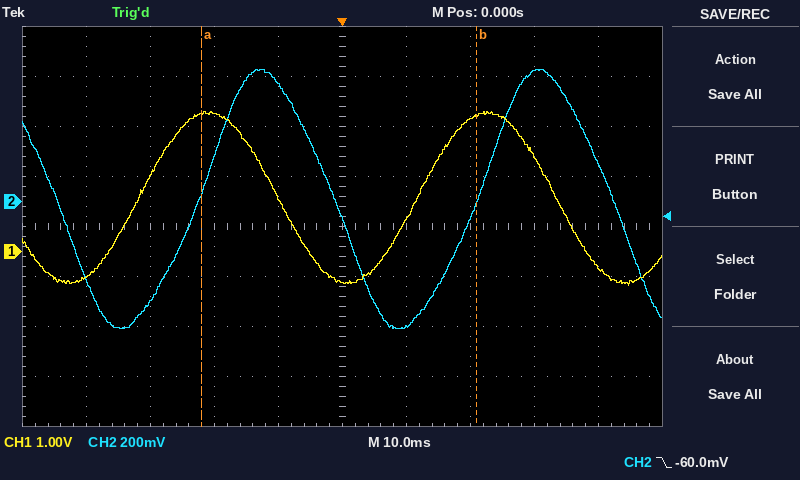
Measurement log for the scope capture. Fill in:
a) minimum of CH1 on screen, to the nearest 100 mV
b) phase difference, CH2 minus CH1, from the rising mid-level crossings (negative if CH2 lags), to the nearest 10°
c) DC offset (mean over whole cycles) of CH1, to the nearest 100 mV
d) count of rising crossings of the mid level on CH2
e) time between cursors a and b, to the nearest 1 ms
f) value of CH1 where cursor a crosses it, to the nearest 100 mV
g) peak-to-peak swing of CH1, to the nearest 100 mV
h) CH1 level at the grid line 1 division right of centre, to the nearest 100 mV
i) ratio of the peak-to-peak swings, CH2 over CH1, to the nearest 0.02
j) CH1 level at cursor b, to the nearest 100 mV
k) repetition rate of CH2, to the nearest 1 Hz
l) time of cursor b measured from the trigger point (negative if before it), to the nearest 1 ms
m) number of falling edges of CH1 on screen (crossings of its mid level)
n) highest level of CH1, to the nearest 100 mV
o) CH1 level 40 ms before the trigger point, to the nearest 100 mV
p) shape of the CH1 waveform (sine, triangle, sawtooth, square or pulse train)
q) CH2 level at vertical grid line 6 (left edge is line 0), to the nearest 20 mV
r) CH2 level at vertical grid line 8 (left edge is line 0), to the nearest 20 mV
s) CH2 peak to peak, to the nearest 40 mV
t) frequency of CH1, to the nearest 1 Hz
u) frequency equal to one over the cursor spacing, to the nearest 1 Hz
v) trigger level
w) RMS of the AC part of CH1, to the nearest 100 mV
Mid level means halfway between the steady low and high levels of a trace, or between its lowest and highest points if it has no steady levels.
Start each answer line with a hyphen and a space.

- -700 mV
- -80°
- 1.1 V
- 2
- 43 ms
- 2.8 V
- 3.5 V
- 600 mV
- 0.30
- 2.7 V
- 23 Hz
- +21 ms
- 2
- 2.8 V
- -500 mV
- sine
- -500 mV
- 520 mV
- 1.04 V
- 23 Hz
- 23 Hz
- -60.0 mV
- 1.2 V
